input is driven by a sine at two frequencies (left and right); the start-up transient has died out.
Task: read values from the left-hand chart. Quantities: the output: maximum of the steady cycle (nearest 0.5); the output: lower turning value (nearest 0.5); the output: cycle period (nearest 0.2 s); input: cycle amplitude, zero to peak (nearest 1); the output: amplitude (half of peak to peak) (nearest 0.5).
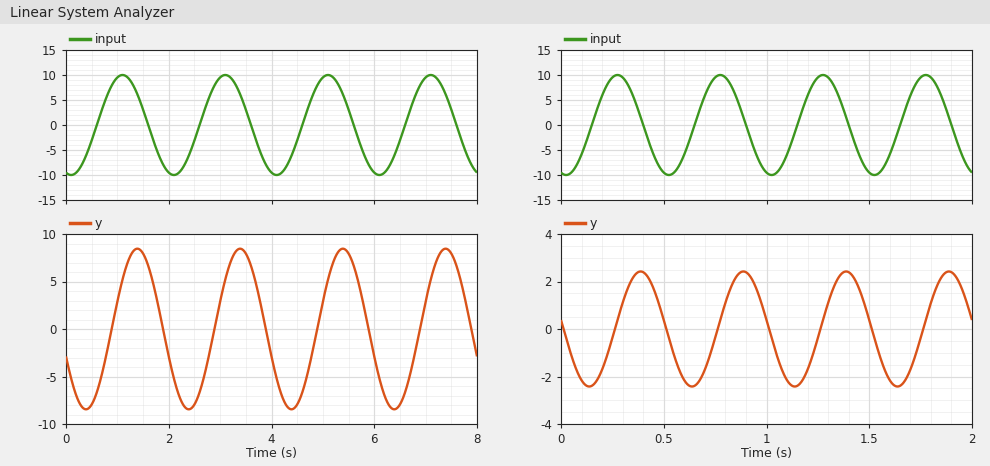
8.5
-8.5
2.0 s
10
8.5
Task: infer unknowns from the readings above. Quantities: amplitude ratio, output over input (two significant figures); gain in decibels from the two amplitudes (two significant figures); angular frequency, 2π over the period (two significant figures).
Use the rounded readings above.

0.85
-1.4 dB
3.1 rad/s
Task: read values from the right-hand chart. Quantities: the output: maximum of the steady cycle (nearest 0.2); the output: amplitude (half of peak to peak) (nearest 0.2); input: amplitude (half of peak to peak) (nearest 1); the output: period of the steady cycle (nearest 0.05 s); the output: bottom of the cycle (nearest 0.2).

2.4
2.4
10
0.50 s
-2.4
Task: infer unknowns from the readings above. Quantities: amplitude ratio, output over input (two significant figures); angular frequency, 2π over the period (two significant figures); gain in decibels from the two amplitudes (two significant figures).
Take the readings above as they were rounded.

0.24
13 rad/s
-12 dB
